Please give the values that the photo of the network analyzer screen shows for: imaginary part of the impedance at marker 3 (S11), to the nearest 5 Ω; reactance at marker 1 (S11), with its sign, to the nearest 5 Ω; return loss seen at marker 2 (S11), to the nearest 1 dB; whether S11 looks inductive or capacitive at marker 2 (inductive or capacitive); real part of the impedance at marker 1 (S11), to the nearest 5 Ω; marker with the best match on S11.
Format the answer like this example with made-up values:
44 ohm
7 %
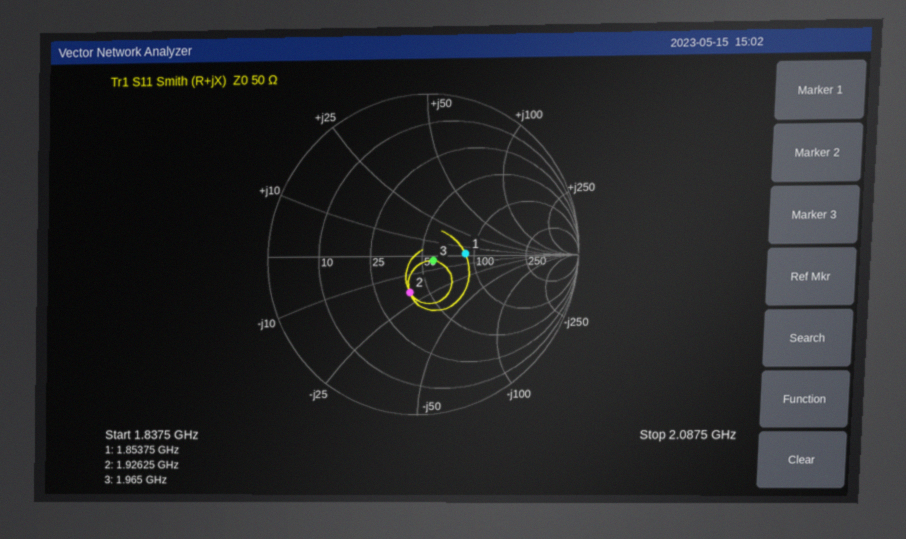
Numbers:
-5 Ω
0 Ω
12 dB
capacitive
90 Ω
marker 3
